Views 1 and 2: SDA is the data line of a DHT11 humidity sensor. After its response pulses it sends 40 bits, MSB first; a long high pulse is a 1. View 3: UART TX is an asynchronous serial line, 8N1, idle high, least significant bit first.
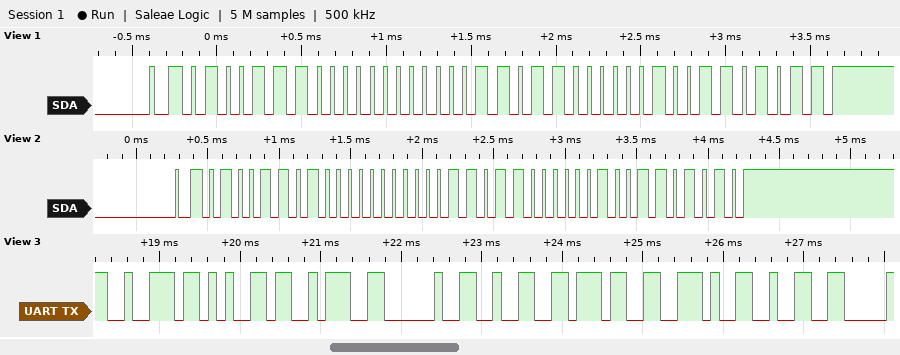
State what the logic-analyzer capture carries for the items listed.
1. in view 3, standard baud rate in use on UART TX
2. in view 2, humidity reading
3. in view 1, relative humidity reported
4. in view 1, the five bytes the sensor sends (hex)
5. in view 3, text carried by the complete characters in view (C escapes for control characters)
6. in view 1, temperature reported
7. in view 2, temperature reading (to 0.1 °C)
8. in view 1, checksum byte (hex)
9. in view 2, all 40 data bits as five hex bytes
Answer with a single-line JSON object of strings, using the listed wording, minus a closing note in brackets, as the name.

{"in view 3, standard baud rate in use on UART TX": "9600 baud", "in view 2, humidity reading": "77 %", "in view 1, relative humidity reported": "78 %", "in view 1, the five bytes the sensor sends": "4E 00 1B 02 6B", "in view 3, text carried by the complete characters in view": "\"re: 27.2\"", "in view 1, temperature reported": "27.2 °C", "in view 2, temperature reading": "27.2 °C", "in view 1, checksum byte": "0x6B", "in view 2, all 40 data bits as five hex bytes": "4D 00 1B 02 6A"}
